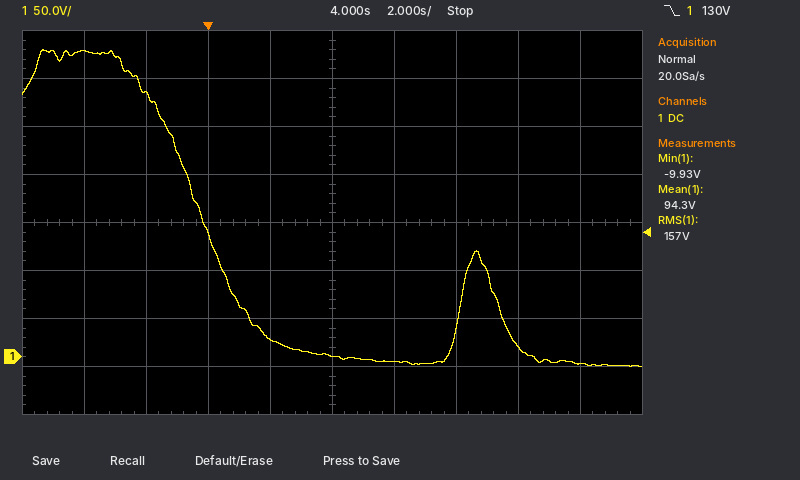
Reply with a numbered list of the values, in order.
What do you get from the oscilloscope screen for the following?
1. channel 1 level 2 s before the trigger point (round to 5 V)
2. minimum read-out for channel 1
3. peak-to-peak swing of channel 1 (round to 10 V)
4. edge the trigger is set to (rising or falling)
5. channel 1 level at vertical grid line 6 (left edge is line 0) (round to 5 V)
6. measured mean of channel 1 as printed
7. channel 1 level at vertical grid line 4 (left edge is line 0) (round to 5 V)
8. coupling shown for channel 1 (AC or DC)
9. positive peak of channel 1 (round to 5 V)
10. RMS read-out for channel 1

1. 275 V
2. -9.93 V
3. 330 V
4. falling
5. -5 V
6. 94.3 V
7. 20 V
8. DC
9. 320 V
10. 157 V
